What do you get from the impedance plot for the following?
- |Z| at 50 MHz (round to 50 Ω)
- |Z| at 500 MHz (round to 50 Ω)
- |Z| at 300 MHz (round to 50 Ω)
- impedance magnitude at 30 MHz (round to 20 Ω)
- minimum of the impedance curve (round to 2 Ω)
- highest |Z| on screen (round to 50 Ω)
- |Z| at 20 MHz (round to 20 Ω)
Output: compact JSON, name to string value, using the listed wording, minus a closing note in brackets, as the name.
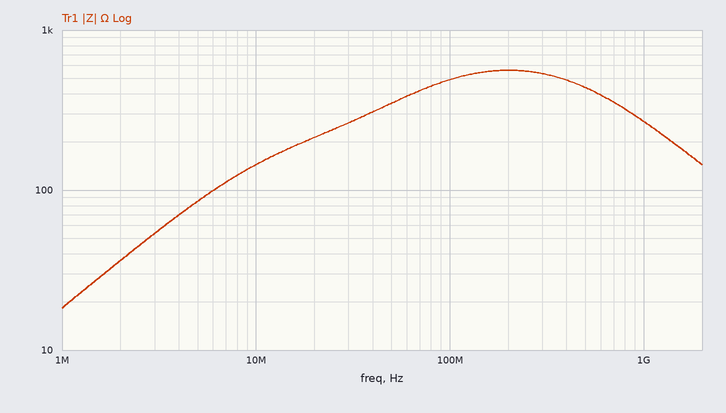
{"|Z| at 50 MHz": "350 Ω", "|Z| at 500 MHz": "450 Ω", "|Z| at 300 MHz": "550 Ω", "impedance magnitude at 30 MHz": "260 Ω", "minimum of the impedance curve": "18 Ω", "highest |Z| on screen": "550 Ω", "|Z| at 20 MHz": "220 Ω"}
